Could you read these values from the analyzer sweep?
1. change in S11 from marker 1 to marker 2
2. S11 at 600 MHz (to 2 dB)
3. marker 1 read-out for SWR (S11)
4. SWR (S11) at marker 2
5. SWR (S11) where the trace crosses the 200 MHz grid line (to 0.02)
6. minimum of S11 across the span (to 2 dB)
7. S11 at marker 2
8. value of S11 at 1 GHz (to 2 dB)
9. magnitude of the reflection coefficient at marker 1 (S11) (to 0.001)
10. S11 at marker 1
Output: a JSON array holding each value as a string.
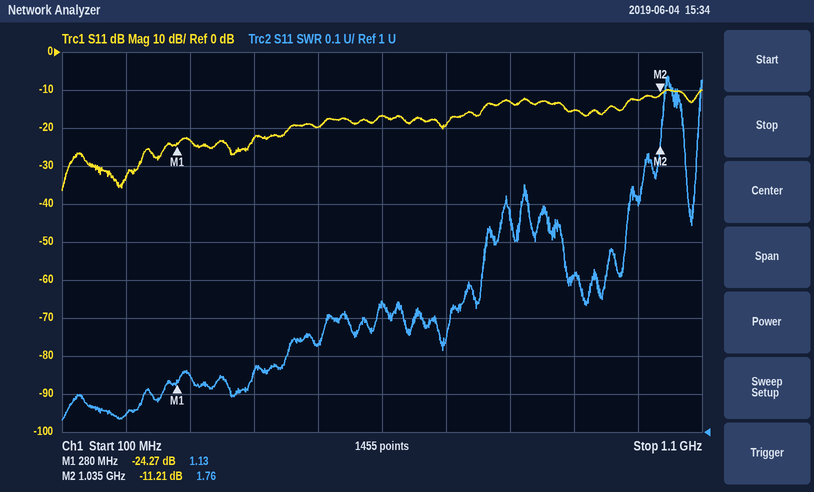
["13.06 dB", "-16 dB", "1.13", "1.76", "1.04", "-36 dB", "-11.21 dB", "-12 dB", "0.061", "-24.27 dB"]
